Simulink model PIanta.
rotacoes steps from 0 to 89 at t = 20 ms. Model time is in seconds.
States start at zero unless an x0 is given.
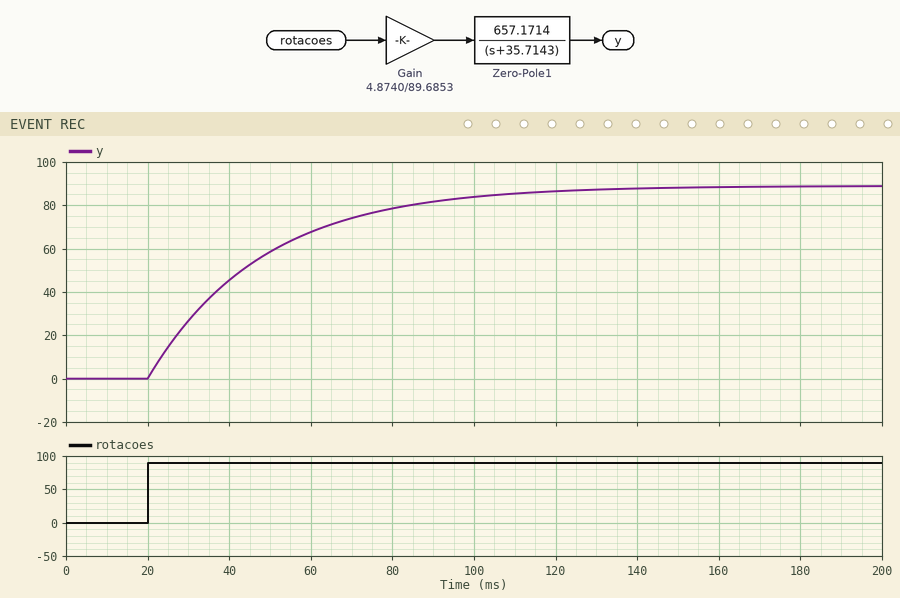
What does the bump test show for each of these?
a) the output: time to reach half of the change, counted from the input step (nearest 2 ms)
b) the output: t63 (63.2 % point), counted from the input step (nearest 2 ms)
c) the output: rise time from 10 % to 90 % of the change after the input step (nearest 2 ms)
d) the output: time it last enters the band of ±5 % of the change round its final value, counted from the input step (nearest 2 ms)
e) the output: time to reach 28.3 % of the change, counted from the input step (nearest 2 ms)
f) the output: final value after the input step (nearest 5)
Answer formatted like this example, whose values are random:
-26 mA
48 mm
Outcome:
20 ms
28 ms
62 ms
84 ms
10 ms
90
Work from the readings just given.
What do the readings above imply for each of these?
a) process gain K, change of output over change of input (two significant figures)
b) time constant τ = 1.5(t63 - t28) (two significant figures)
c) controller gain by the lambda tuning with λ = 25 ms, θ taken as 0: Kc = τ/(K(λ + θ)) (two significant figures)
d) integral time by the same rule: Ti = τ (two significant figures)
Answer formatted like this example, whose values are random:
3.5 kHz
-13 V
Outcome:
1.0
27 ms
1.1
27 ms
